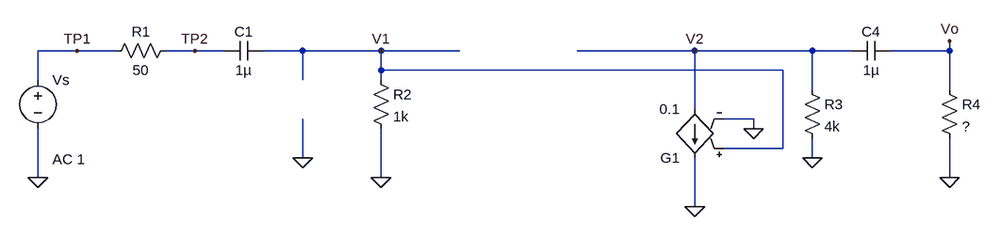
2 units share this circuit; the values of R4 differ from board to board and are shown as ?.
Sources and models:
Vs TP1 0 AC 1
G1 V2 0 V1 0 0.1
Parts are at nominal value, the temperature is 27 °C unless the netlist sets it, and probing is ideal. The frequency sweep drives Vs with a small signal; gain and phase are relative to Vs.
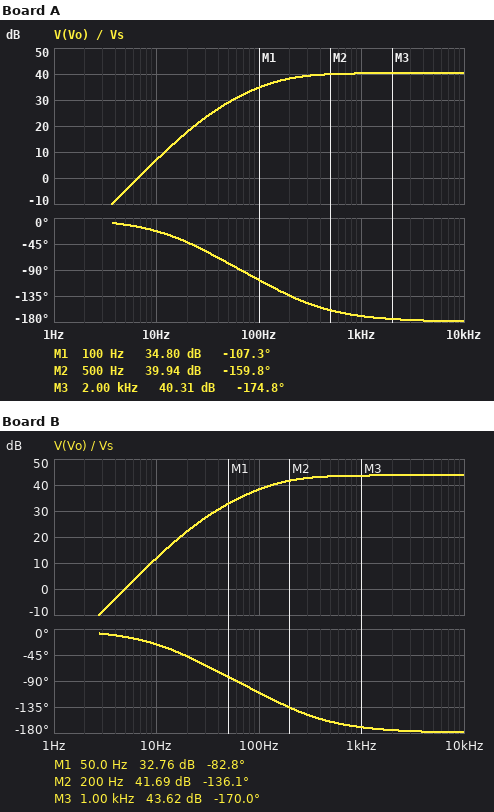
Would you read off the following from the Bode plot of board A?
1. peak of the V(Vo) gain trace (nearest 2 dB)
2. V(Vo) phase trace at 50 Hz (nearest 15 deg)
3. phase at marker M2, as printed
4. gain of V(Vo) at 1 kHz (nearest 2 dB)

40 dB
-75 deg
-159.8 deg
40 dB
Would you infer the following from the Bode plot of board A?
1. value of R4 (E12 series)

1.5 kΩ
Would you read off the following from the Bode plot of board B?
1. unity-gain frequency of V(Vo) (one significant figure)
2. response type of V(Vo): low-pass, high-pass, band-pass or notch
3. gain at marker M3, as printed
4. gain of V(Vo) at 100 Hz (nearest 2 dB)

5 Hz
high-pass
43.62 dB
38 dB
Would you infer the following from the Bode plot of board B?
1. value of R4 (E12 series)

2.7 kΩ
